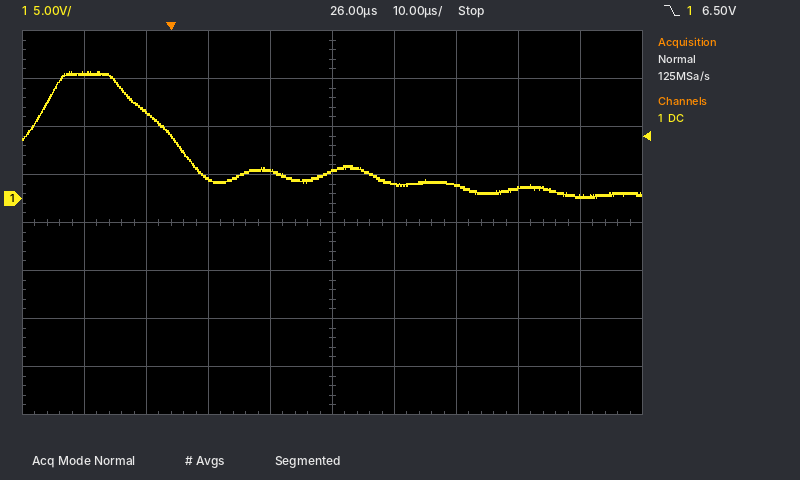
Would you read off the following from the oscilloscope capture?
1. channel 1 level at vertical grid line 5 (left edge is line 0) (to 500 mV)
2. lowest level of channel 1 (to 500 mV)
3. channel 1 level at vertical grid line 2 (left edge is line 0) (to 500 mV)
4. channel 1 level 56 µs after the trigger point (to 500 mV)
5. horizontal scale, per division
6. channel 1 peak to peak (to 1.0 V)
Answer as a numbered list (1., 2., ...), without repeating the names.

1. 3.0 V
2. 0.0 V
3. 9.0 V
4. 1.0 V
5. 10 µs
6. 13.0 V
